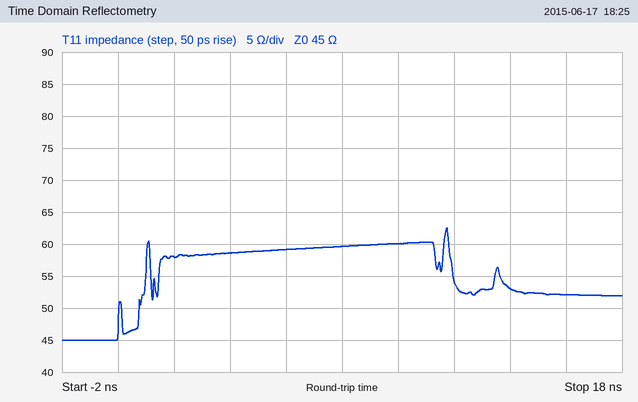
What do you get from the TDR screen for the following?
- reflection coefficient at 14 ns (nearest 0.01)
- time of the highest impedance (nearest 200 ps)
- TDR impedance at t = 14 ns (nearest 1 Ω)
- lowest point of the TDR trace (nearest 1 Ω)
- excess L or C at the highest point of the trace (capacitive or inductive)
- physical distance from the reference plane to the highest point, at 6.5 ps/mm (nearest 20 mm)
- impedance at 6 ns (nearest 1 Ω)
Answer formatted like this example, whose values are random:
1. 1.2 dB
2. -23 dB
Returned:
1. +0.08
2. 11.8 ns
3. 53 Ω
4. 45 Ω
5. inductive
6. 900 mm
7. 59 Ω
